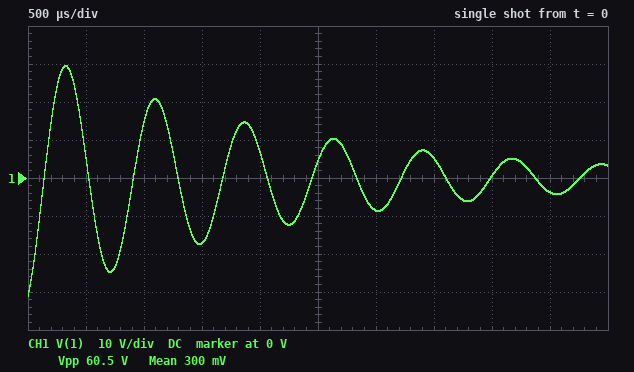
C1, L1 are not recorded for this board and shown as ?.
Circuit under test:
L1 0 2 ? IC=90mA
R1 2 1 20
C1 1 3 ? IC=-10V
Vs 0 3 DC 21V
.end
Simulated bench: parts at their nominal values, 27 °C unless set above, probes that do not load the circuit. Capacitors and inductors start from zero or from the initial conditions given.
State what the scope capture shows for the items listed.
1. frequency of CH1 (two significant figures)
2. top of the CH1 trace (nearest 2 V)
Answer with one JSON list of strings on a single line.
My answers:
["1.3 kHz", "30 V"]
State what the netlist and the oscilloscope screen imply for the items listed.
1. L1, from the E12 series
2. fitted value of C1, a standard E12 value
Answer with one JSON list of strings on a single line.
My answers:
["22 mH", "680 nF"]
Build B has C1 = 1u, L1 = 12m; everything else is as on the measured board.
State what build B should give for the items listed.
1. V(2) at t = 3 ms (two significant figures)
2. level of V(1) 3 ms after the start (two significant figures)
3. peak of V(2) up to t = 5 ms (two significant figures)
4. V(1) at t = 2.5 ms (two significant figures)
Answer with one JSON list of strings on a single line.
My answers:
["2.2 V", "1.9 V", "25 V", "2.3 V"]
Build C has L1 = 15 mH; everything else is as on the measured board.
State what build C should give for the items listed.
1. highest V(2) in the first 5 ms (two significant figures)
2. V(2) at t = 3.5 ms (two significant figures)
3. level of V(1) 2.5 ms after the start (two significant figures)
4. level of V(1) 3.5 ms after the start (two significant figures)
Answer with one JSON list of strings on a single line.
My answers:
["28 V", "2.8 V", "-6.2 V", "3.0 V"]
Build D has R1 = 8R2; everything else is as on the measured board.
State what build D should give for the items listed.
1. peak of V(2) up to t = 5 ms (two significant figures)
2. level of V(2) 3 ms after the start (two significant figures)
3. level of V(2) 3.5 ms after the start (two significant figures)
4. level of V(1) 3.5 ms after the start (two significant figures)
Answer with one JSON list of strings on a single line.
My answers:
["33 V", "-20 V", "12 V", "13 V"]
